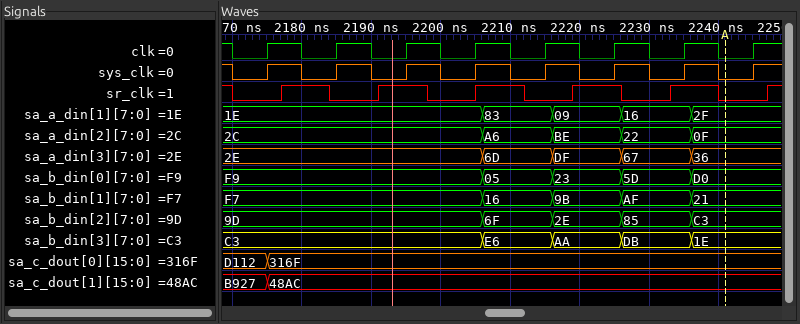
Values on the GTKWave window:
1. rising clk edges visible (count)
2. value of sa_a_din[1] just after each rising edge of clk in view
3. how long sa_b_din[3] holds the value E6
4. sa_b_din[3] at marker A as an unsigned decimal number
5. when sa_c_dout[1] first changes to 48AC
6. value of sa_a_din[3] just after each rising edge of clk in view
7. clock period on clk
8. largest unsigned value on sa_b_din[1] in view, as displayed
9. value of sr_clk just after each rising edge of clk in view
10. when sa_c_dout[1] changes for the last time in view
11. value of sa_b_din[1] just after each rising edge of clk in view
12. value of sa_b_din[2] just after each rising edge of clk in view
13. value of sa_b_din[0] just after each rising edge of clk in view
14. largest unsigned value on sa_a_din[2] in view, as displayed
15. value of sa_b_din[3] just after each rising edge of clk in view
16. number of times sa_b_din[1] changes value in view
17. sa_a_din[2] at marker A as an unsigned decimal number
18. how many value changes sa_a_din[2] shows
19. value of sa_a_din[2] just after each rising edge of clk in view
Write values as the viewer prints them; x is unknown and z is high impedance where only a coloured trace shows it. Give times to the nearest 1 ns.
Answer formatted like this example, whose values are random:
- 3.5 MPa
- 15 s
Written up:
- 8
- 1E, 1E, 1E, 1E, 83, 09, 16, 2F
- 10 ns
- 30
- 2175 ns
- 2E, 2E, 2E, 2E, 6D, DF, 67, 36
- 10 ns
- F7
- 0 0 1 1 0 1 1 0
- 2175 ns
- F7, F7, F7, F7, 16, 9B, AF, 21
- 9D, 9D, 9D, 9D, 6F, 2E, 85, C3
- F9, F9, F9, F9, 05, 23, 5D, D0
- BE
- C3, C3, C3, C3, E6, AA, DB, 1E
- 4
- 15
- 4
- 2C, 2C, 2C, 2C, A6, BE, 22, 0F
